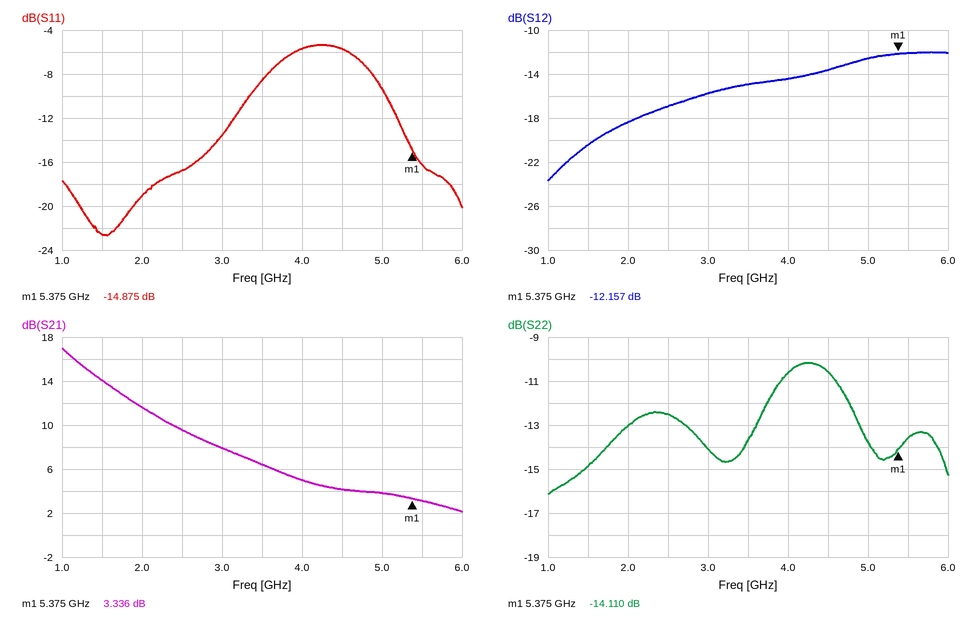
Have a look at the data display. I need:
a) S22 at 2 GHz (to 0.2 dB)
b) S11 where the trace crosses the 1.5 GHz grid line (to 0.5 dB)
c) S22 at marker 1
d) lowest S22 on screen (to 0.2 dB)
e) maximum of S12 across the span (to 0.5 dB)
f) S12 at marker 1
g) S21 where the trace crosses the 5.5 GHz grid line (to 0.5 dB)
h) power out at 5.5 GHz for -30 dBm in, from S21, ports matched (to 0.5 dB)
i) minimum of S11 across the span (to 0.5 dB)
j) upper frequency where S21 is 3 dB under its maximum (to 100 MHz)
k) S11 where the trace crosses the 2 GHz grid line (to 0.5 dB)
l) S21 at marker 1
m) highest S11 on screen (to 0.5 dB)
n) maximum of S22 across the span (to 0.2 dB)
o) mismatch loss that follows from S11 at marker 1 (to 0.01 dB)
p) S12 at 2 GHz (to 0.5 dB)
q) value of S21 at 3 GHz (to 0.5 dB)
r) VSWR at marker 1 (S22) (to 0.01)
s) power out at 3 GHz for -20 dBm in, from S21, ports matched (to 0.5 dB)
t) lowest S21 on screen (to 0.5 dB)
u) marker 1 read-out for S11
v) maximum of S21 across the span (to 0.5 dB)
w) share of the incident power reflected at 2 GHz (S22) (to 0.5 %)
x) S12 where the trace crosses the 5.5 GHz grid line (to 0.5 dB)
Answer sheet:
-13.0 dB
-22.5 dB
-14.110 dB
-16.2 dB
-12.0 dB
-12.157 dB
3.0 dB
-27.0 dBm
-22.5 dB
1.5 GHz
-19.0 dB
3.336 dB
-5.5 dB
-10.2 dB
0.14 dB
-18.5 dB
8.0 dB
1.49
-12.0 dBm
2.0 dB
-14.875 dB
17.0 dB
5.0 %
-12.0 dB
